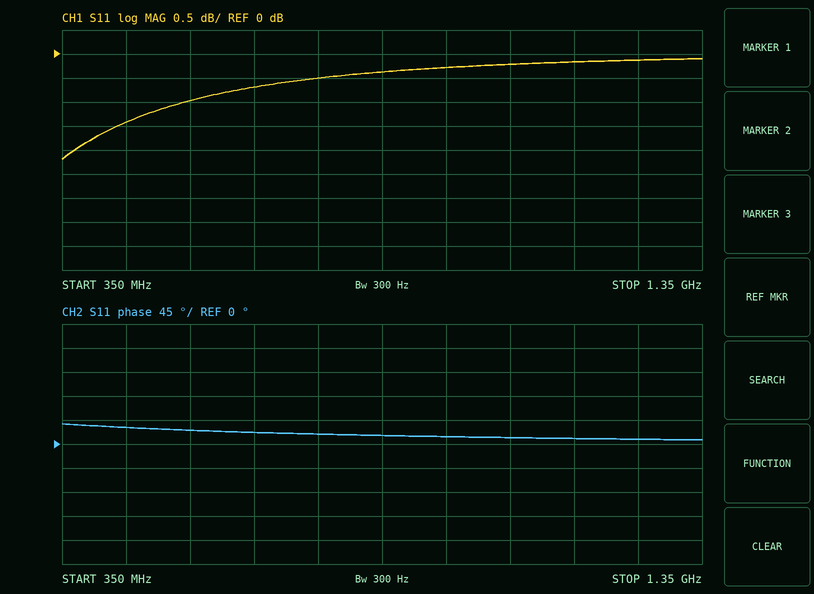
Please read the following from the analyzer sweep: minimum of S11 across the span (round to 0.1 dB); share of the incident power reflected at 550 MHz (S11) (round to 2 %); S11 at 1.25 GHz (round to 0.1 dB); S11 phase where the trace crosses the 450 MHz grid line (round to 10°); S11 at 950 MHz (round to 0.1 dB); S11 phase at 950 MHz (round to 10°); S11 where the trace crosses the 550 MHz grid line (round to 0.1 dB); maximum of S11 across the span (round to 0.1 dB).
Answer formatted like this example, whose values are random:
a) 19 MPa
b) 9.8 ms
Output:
a) -2.2 dB
b) 80 %
c) -0.1 dB
d) 30°
e) -0.3 dB
f) 10°
g) -1.0 dB
h) -0.1 dB
